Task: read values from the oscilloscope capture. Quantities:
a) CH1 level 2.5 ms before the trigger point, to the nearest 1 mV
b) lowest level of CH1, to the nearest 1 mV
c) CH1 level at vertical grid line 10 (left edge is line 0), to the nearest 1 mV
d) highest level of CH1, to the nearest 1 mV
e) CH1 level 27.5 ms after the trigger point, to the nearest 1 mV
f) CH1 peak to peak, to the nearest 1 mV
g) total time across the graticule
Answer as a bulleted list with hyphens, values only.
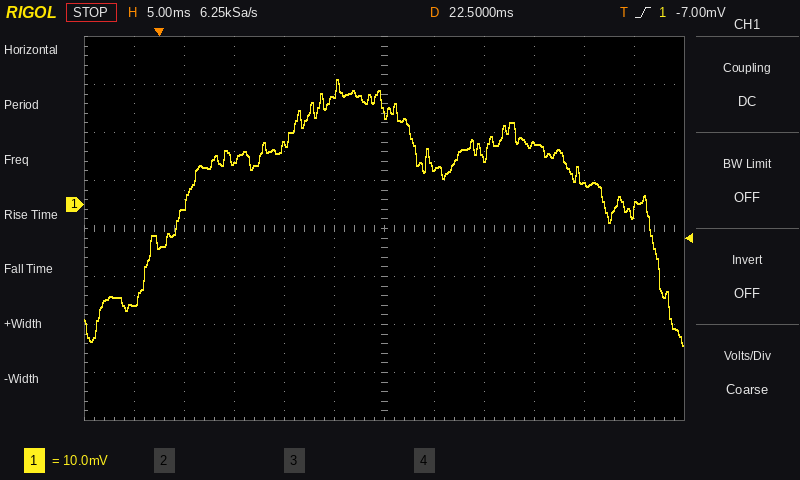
- -21 mV
- -29 mV
- 4 mV
- 26 mV
- 8 mV
- 55 mV
- 60 ms
